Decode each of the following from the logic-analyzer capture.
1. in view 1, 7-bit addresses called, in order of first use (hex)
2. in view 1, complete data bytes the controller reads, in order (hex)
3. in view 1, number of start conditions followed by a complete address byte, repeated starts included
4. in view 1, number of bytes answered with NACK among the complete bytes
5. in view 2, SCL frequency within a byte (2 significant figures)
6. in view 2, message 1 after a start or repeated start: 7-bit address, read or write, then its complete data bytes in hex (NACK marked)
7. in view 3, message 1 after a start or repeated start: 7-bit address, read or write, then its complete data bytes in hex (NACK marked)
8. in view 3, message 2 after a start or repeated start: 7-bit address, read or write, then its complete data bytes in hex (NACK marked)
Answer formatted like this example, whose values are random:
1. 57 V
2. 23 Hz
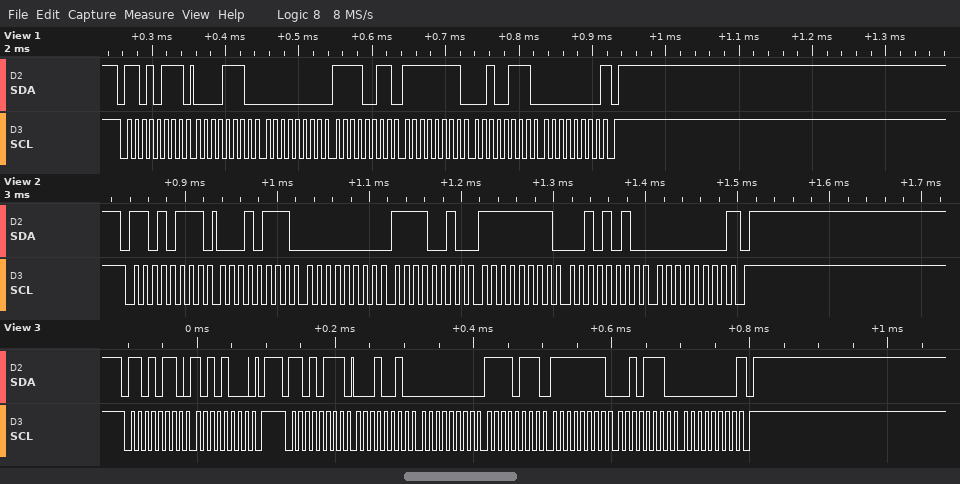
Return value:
1. 0x6B
2. 0E 00 F3 FF 27 00
3. 1
4. 1
5. 100 kHz
6. 0x6B read: 17 00 F2 FF 2A 00 NACK
7. 0x6B write: A8
8. 0x6B read: 12 00 F7 FF 2E 00 NACK
